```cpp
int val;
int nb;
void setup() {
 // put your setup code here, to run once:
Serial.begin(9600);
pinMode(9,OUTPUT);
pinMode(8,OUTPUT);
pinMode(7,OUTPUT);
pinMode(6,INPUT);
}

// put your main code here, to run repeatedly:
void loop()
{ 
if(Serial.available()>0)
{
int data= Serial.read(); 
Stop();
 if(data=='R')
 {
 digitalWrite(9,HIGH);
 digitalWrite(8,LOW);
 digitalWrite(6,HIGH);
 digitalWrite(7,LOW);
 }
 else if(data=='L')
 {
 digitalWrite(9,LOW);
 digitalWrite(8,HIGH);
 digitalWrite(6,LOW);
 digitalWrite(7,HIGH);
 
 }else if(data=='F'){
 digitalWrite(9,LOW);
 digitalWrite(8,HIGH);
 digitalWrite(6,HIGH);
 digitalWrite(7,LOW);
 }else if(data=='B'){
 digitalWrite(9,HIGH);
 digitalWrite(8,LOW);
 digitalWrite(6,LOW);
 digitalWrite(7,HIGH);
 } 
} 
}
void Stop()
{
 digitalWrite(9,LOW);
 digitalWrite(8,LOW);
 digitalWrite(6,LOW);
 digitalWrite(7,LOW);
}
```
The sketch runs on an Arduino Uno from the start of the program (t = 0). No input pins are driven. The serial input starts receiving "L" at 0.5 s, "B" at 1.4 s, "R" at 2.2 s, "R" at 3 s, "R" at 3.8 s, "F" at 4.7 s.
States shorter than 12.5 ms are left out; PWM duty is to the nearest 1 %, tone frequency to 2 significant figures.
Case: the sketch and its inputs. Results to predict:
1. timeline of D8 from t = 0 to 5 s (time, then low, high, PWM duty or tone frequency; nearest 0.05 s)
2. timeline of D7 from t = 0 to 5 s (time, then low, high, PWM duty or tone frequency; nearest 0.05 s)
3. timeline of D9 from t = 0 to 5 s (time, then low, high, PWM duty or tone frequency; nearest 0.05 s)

0 s low; 0.5 s high; 1.4 s low; 4.7 s high
0 s low; 0.5 s high; 2.2 s low
0 s low; 1.4 s high; 4.7 s low
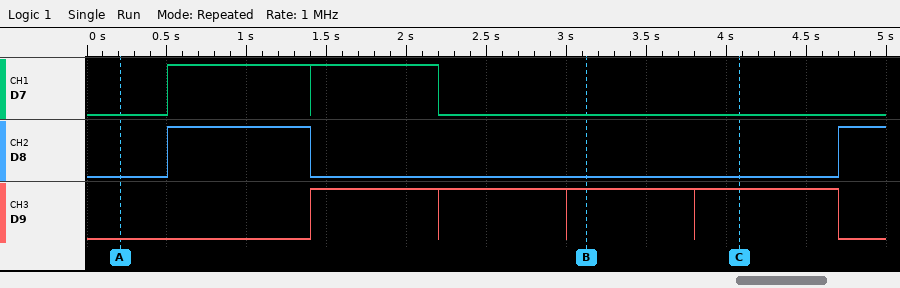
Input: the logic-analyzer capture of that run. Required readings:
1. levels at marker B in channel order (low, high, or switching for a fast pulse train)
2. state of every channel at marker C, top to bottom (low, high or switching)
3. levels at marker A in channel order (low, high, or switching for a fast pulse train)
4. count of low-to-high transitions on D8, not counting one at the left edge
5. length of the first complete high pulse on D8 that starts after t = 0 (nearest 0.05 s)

D7 low, D8 low, D9 high
D7 low, D8 low, D9 high
D7 low, D8 low, D9 low
2
0.90 s
